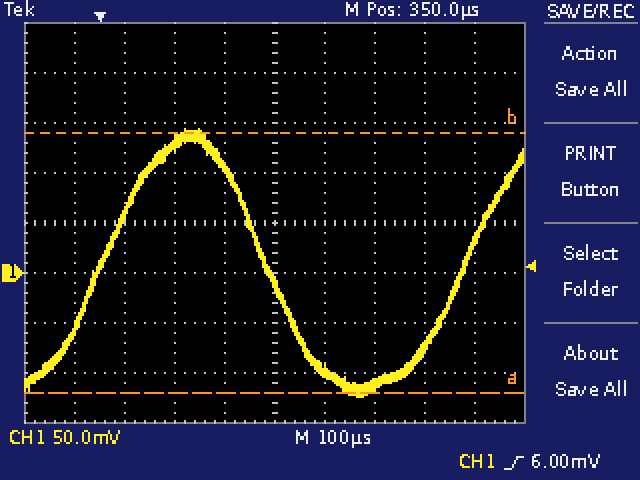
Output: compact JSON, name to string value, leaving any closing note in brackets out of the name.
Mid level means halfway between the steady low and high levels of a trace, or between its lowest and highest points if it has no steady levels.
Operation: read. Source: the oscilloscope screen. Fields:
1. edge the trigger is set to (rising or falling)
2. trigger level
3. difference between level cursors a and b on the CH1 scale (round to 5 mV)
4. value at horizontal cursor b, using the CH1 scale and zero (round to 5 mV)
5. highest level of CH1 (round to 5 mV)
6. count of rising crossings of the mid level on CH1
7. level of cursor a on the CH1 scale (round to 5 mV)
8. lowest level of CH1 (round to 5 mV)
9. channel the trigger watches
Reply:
{"edge the trigger is set to": "rising", "trigger level": "6.00 mV", "difference between level cursors a and b on the CH1 scale": "260 mV", "value at horizontal cursor b, using the CH1 scale and zero": "140 mV", "highest level of CH1": "145 mV", "count of rising crossings of the mid level on CH1": "2", "level of cursor a on the CH1 scale": "-120 mV", "lowest level of CH1": "-125 mV", "channel the trigger watches": "CH1"}
